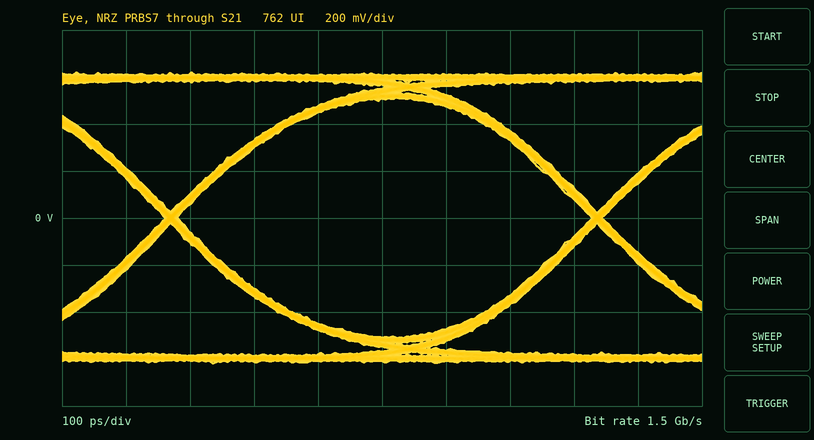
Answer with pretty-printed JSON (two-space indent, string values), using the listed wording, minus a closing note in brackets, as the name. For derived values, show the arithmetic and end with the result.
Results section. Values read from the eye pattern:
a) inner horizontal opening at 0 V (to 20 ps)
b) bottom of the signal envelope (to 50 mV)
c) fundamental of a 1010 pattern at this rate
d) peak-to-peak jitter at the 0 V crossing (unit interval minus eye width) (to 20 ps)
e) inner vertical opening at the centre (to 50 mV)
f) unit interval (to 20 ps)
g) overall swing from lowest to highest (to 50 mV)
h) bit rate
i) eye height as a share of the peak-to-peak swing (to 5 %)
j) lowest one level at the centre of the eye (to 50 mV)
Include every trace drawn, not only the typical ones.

{
  "inner horizontal opening at 0 V": "640 ps",
  "bottom of the signal envelope": "-600 mV",
  "fundamental of a 1010 pattern at this rate": "750 MHz",
  "peak-to-peak jitter at the 0 V crossing (unit interval minus eye width)": "20 ps",
  "inner vertical opening at the centre": "1.00 V",
  "unit interval": "660 ps",
  "overall swing from lowest to highest": "1.25 V",
  "bit rate": "1.5 Gb/s",
  "eye height as a share of the peak-to-peak swing": "1.00 V / 1.25 V ≈ 80 %",
  "lowest one level at the centre of the eye": "500 mV"
}
